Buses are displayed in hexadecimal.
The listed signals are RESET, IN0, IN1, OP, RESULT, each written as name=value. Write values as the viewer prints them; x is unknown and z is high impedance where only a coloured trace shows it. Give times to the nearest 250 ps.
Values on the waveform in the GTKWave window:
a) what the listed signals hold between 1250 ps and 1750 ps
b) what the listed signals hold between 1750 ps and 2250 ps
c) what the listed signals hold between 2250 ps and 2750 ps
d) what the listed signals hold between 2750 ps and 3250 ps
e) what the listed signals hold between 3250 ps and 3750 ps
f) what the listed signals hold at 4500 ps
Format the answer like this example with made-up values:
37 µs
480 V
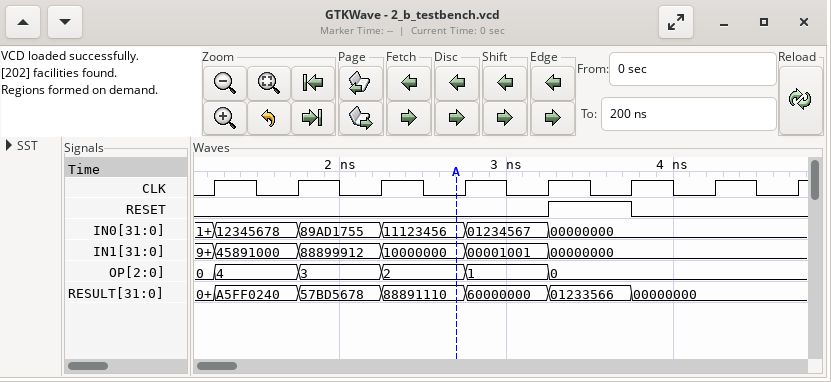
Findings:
RESET=0, IN0=12345678, IN1=45891000, OP=4, RESULT=A5FF0240
RESET=0, IN0=89AD1755, IN1=88899912, OP=3, RESULT=57BD5678
RESET=0, IN0=11123456, IN1=10000000, OP=2, RESULT=88891110
RESET=0, IN0=01234567, IN1=00001001, OP=1, RESULT=60000000
RESET=1, IN0=00000000, IN1=00000000, OP=0, RESULT=01233566
RESET=0, IN0=00000000, IN1=00000000, OP=0, RESULT=00000000
